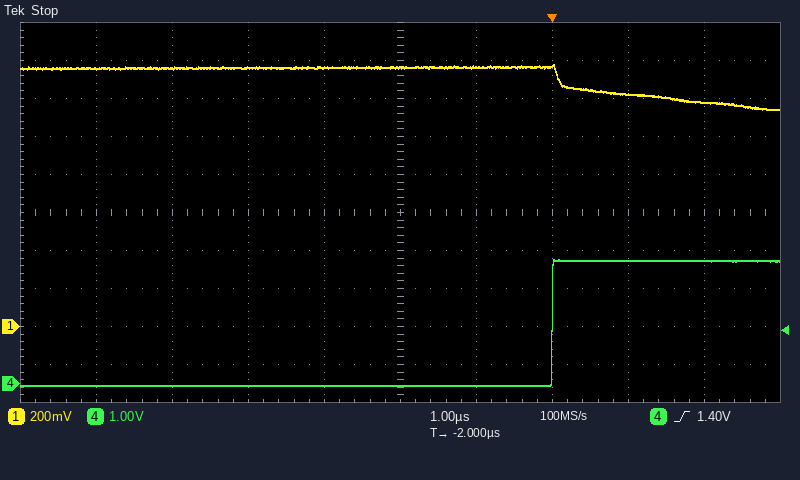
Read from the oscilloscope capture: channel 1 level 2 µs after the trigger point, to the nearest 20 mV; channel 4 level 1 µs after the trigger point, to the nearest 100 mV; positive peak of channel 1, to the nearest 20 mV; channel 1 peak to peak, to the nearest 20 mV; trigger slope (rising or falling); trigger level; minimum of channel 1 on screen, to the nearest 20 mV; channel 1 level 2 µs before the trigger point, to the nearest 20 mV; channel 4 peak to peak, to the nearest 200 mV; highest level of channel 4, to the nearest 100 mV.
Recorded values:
1.18 V
3.2 V
1.38 V
240 mV
rising
1.40 V
1.14 V
1.36 V
3.4 V
3.3 V
